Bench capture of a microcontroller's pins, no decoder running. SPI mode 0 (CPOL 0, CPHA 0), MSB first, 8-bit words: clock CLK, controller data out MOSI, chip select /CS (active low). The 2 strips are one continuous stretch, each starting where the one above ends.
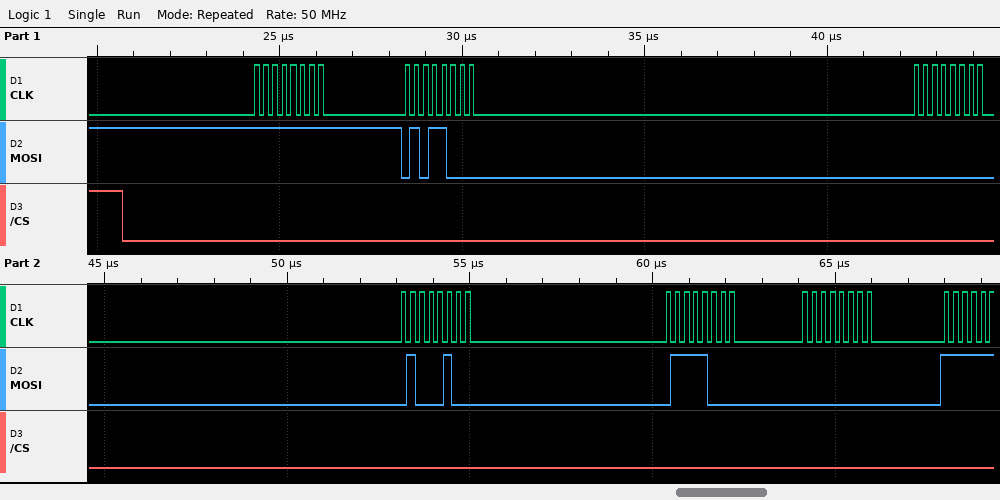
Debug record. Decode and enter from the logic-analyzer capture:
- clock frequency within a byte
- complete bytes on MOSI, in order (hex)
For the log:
4 MHz
FF 58 00 44 78 00
